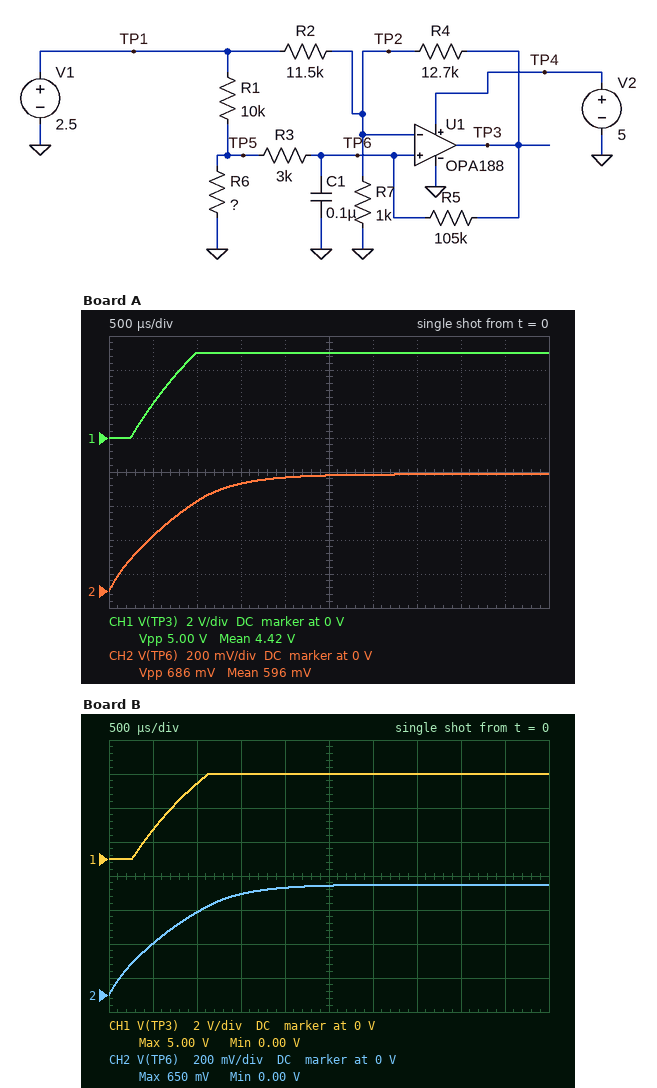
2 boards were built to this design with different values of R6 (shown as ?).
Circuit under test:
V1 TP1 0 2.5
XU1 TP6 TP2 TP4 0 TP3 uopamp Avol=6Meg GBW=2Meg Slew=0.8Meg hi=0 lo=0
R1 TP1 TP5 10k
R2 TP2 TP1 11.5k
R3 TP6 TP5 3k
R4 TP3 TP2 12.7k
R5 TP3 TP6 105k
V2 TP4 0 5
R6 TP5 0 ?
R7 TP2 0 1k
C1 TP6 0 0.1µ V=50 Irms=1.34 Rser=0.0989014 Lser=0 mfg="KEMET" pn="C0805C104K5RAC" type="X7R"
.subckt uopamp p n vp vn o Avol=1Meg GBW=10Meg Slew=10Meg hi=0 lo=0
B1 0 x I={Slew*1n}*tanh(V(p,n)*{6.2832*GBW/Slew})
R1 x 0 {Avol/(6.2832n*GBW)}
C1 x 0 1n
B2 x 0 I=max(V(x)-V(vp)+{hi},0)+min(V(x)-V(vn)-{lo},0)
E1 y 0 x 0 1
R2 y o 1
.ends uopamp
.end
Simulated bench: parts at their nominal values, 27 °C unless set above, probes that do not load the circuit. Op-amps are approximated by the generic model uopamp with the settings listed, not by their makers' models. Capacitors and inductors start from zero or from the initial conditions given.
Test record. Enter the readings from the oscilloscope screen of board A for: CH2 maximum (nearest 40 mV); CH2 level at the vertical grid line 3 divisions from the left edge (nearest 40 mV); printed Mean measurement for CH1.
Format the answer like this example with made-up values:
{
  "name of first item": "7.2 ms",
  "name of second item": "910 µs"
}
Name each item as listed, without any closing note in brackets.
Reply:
{
  "CH2 maximum": "680 mV",
  "CH2 level at the vertical grid line 3 divisions from the left edge": "640 mV",
  "printed Mean measurement for CH1": "4.42 V"
}
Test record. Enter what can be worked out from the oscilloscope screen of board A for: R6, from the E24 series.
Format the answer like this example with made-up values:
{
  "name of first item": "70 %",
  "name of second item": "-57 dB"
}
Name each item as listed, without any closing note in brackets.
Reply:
{
  "R6, from the E24 series": "2.4 kΩ"
}
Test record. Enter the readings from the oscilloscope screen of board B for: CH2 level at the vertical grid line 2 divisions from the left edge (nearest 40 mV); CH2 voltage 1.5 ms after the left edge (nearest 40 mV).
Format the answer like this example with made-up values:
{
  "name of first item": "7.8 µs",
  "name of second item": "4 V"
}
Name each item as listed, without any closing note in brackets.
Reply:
{
  "CH2 level at the vertical grid line 2 divisions from the left edge": "480 mV",
  "CH2 voltage 1.5 ms after the left edge": "600 mV"
}
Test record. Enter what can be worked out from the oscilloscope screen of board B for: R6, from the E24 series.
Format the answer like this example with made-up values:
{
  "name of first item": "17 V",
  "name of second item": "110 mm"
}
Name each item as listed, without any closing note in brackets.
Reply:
{
  "R6, from the E24 series": "2.2 kΩ"
}
